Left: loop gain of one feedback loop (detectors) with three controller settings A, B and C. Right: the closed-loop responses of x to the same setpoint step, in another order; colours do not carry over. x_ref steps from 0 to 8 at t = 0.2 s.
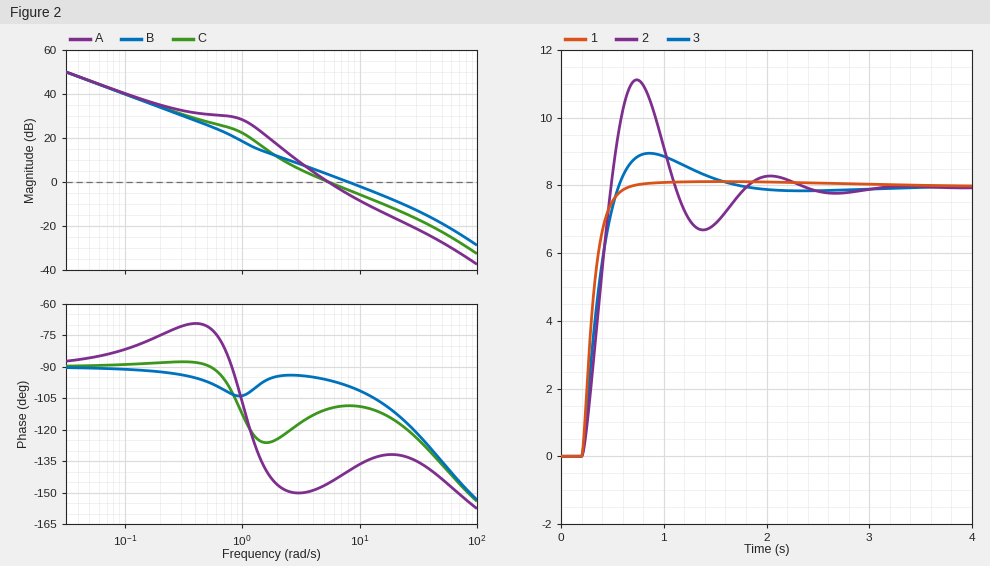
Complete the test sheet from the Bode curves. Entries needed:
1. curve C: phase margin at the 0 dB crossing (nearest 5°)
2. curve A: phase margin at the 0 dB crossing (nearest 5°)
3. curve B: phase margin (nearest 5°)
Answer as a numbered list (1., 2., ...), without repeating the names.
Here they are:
1. 70°
2. 35°
3. 80°
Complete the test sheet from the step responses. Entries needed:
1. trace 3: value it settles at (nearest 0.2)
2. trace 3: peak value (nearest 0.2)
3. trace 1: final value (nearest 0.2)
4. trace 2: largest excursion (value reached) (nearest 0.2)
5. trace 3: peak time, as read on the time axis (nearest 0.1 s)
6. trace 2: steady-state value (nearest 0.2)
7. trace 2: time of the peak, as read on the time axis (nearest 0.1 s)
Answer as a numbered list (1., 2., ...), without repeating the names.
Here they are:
1. 8.0
2. 9.0
3. 8.0
4. 11.2
5. 0.9 s
6. 8.0
7. 0.7 s
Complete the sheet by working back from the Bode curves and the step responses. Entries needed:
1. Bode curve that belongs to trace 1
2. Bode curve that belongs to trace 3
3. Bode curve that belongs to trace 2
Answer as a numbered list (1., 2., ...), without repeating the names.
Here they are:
1. B
2. C
3. A
